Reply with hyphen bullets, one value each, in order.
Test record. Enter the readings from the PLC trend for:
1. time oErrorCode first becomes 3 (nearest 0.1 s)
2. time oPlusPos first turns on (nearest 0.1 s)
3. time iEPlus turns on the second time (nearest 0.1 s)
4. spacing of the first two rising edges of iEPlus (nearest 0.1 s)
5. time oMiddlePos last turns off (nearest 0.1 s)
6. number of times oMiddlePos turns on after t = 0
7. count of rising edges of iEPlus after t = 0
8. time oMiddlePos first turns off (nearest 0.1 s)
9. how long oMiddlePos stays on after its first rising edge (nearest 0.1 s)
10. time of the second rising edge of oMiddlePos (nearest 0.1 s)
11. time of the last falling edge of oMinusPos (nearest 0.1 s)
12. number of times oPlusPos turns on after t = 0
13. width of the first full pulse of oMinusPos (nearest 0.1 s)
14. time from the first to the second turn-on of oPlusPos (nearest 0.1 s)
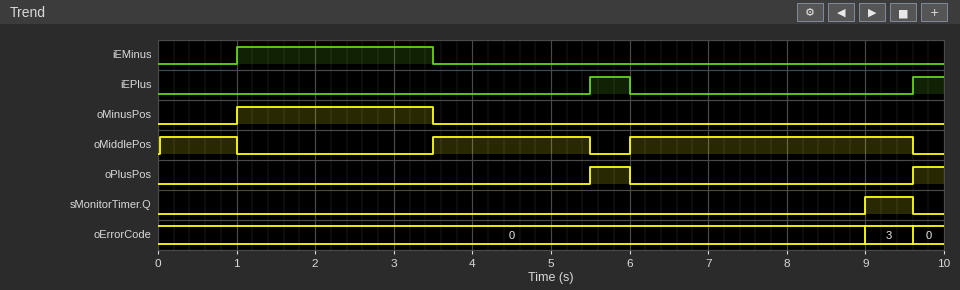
- 9.0 s
- 5.5 s
- 9.6 s
- 4.1 s
- 9.6 s
- 3
- 2
- 1.0 s
- 1.0 s
- 3.5 s
- 3.5 s
- 2
- 2.5 s
- 4.1 s
